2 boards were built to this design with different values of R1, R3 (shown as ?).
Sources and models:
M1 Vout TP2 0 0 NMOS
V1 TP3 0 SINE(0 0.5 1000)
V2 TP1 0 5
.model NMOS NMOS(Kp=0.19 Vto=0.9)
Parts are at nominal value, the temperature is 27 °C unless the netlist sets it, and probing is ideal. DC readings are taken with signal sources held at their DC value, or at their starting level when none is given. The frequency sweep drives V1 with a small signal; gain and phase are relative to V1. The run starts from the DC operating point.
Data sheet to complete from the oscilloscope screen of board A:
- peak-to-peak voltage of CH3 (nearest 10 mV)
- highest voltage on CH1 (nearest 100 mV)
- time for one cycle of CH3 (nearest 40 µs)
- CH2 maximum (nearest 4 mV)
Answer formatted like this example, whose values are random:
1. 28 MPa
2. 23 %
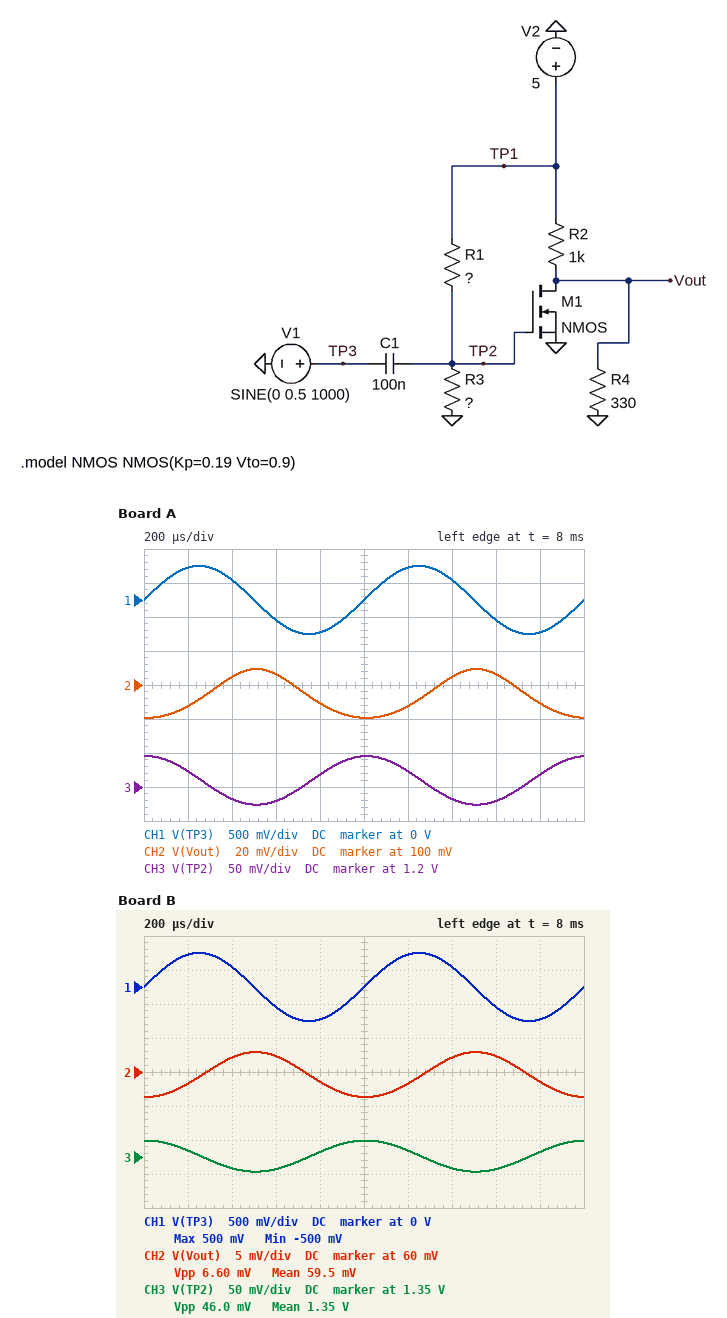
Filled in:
1. 70 mV
2. 500 mV
3. 1.00 ms
4. 108 mV
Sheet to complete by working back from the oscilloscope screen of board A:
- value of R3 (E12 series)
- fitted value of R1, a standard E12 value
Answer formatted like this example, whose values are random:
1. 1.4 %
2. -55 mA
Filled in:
1. 150 Ω
2. 470 Ω
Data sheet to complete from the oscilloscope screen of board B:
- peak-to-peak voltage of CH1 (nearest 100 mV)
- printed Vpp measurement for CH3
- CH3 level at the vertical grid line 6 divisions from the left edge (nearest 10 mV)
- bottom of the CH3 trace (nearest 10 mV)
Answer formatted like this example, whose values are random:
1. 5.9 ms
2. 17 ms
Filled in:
1. 1.0 V
2. 46.0 mV
3. 1.36 V
4. 1.33 V
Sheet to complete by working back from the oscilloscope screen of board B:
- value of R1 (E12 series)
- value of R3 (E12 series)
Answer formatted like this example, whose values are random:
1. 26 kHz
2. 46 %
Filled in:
1. 270 Ω
2. 100 Ω
